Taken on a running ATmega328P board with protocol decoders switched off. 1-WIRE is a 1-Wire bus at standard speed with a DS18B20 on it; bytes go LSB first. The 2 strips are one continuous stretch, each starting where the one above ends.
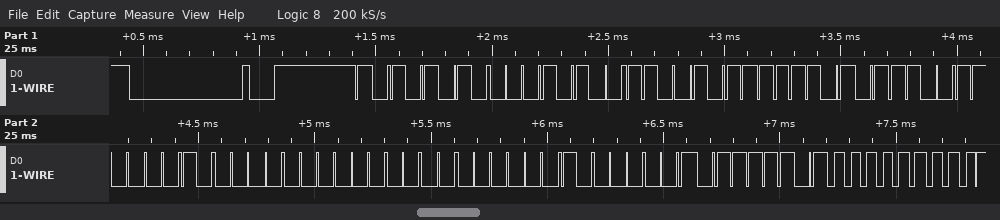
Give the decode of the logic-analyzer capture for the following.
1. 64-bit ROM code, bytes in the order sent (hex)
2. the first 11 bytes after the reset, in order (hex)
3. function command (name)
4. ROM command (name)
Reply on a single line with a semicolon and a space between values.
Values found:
28 D3 AF 33 04 00 00 81; 55 28 D3 AF 33 04 00 00 81 BE 00; Read Scratchpad; Match ROM
